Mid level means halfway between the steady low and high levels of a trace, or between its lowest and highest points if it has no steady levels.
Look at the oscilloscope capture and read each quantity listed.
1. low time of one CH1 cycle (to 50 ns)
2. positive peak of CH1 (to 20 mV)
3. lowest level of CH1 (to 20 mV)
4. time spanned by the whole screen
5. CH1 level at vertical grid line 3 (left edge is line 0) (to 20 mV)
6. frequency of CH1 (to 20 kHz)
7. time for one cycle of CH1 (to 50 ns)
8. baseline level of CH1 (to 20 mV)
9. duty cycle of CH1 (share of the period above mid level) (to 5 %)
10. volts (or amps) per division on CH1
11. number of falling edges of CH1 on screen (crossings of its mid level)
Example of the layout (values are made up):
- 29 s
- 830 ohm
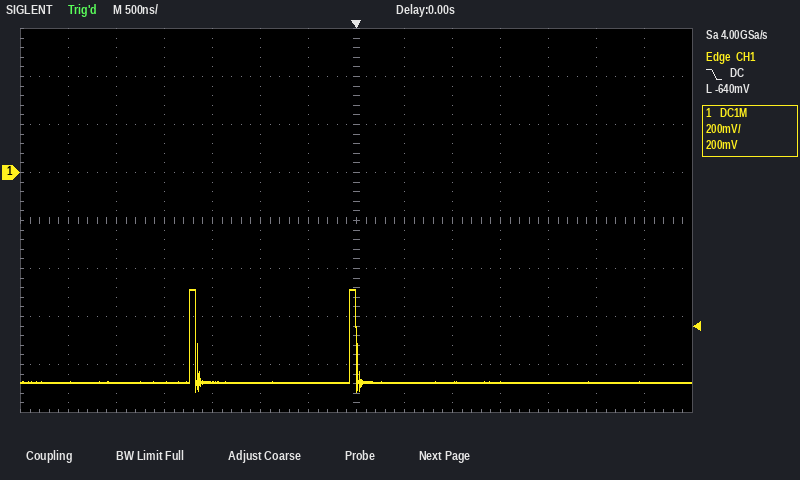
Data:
- 1.60 µs
- -480 mV
- -920 mV
- 7 µs
- -880 mV
- 600 kHz
- 1.65 µs
- -880 mV
- 5 %
- 200 mV
- 2
